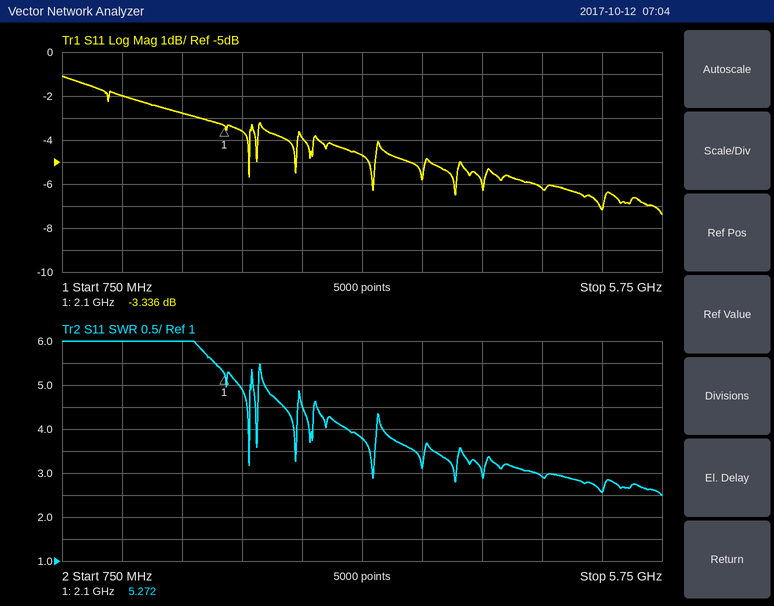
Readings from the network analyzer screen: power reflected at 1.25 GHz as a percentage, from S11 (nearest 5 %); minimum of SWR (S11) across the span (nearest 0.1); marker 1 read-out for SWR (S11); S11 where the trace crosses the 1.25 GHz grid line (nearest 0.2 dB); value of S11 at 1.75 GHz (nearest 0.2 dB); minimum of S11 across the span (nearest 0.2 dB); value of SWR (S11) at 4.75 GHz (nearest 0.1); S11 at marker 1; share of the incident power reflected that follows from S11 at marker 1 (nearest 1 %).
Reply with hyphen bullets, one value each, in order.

- 65 %
- 2.5
- 5.272
- -2.0 dB
- -2.8 dB
- -7.4 dB
- 2.9
- -3.336 dB
- 46 %
